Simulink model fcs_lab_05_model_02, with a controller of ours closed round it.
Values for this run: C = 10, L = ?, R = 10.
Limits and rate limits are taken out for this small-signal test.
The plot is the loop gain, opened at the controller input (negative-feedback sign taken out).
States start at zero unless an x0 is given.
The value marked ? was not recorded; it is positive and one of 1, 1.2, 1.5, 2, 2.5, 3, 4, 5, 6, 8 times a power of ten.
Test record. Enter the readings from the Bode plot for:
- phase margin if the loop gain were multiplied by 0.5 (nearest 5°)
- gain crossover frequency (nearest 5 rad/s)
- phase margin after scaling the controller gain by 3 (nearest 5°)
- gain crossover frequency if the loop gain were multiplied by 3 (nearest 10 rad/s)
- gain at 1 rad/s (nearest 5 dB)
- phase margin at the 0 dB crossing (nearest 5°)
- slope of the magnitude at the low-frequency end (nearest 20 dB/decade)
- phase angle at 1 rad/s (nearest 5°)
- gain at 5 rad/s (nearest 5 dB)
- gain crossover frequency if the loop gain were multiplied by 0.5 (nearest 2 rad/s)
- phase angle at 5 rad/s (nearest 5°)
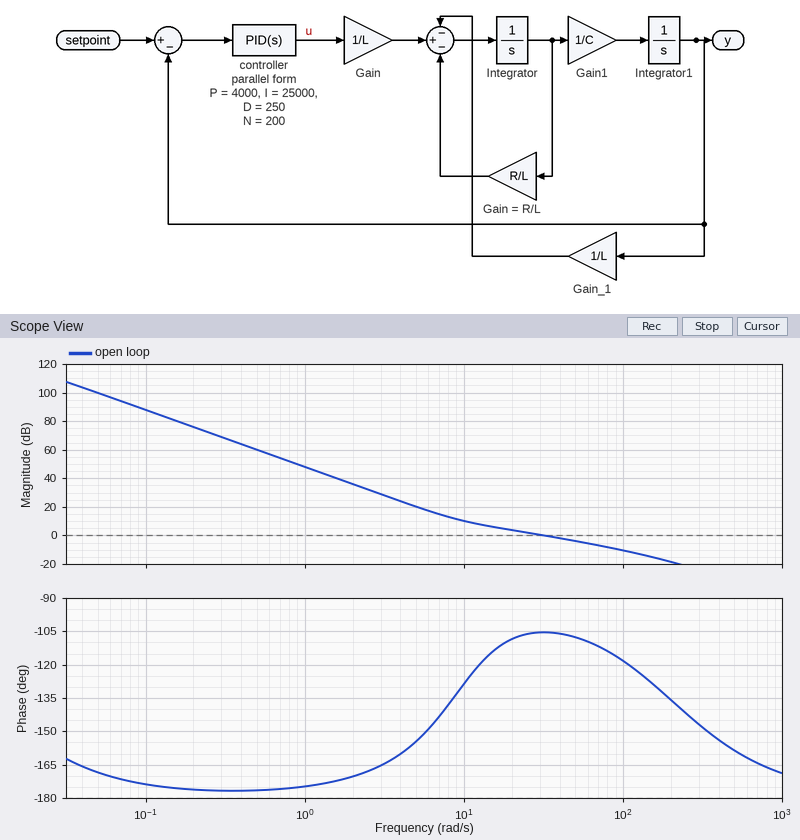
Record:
65°
30 rad/s
65°
90 rad/s
50 dB
75°
-40 dB/decade
-175°
20 dB
16 rad/s
-155°
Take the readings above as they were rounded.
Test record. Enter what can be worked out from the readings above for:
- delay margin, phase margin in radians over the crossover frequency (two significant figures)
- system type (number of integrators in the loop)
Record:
0.044 s
2
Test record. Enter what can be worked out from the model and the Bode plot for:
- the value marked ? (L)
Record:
0.8
